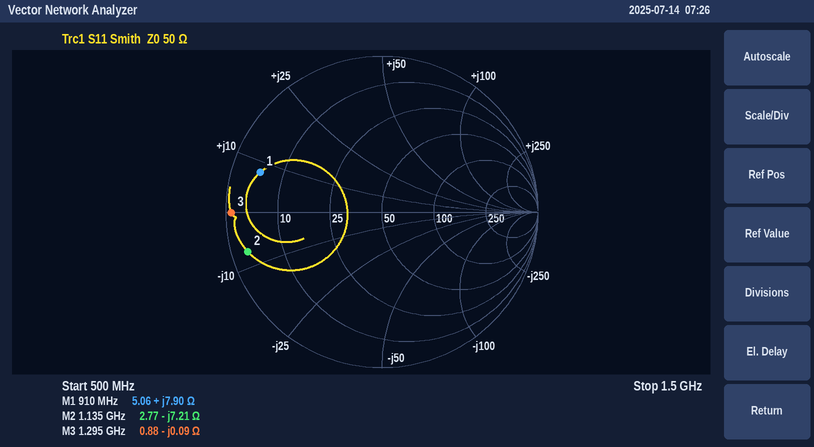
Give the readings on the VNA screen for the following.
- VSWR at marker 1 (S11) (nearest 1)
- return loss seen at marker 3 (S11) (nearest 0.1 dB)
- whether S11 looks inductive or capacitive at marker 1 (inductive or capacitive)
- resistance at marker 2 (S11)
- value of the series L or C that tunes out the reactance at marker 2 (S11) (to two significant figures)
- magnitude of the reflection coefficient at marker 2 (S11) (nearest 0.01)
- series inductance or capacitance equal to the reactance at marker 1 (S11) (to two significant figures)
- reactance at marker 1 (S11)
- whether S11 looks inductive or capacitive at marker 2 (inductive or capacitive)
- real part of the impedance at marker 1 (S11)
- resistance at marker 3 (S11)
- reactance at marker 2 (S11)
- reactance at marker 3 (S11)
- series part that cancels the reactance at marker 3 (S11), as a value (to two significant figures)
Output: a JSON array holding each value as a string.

["10", "0.3 dB", "inductive", "2.77 Ω", "1.0 nH", "0.90", "1.4 nH", "+7.90 Ω", "capacitive", "5.06 Ω", "0.88 Ω", "-7.21 Ω", "-0.09 Ω", "11 pH"]
